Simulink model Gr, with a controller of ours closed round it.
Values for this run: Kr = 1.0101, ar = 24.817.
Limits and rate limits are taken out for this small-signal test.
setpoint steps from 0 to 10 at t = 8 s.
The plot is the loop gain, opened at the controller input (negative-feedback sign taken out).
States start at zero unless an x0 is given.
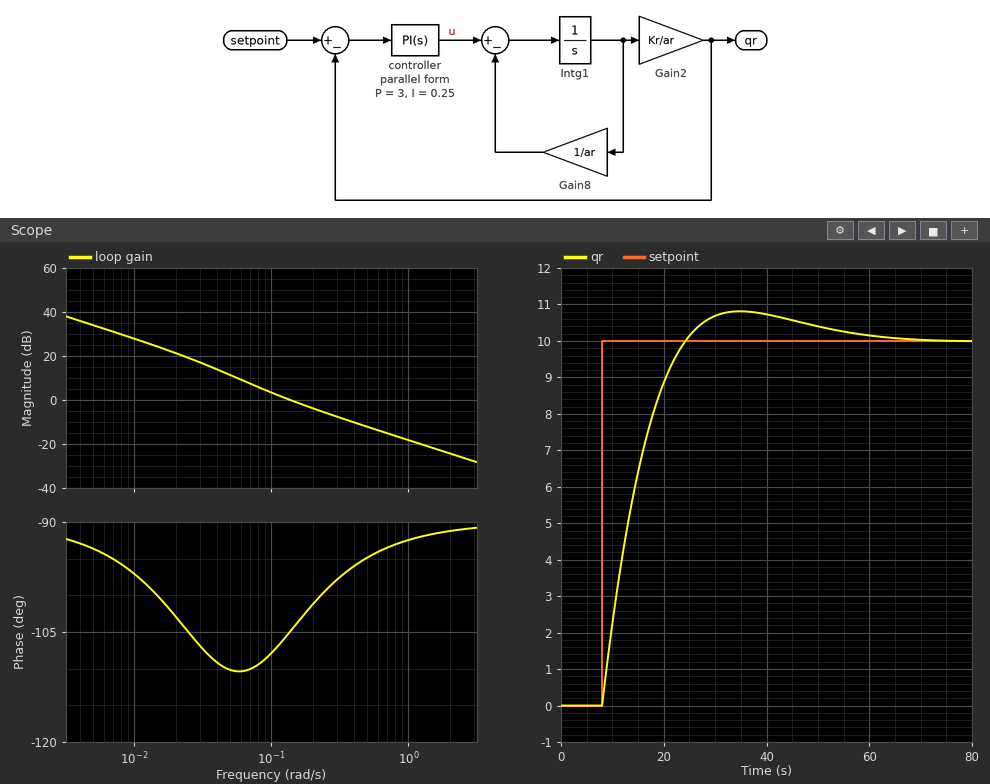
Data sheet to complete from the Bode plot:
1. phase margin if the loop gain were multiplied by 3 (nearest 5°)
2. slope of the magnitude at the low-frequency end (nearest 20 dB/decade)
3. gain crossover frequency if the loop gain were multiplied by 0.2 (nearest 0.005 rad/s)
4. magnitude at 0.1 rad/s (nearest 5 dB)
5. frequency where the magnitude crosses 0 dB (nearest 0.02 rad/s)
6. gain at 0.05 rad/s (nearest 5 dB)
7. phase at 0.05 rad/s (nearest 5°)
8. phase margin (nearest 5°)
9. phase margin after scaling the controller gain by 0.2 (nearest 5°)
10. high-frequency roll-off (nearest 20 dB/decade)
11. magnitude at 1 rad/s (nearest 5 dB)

85°
-20 dB/decade
0.040 rad/s
5 dB
0.14 rad/s
10 dB
-110°
75°
70°
-20 dB/decade
-20 dB
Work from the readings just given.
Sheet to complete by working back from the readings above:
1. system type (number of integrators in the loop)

1
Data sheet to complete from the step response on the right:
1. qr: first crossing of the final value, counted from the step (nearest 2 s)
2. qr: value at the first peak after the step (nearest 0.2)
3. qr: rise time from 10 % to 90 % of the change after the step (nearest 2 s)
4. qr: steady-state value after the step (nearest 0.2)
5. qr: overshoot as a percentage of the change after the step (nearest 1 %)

16 s
10.8
12 s
10.0
8 %
